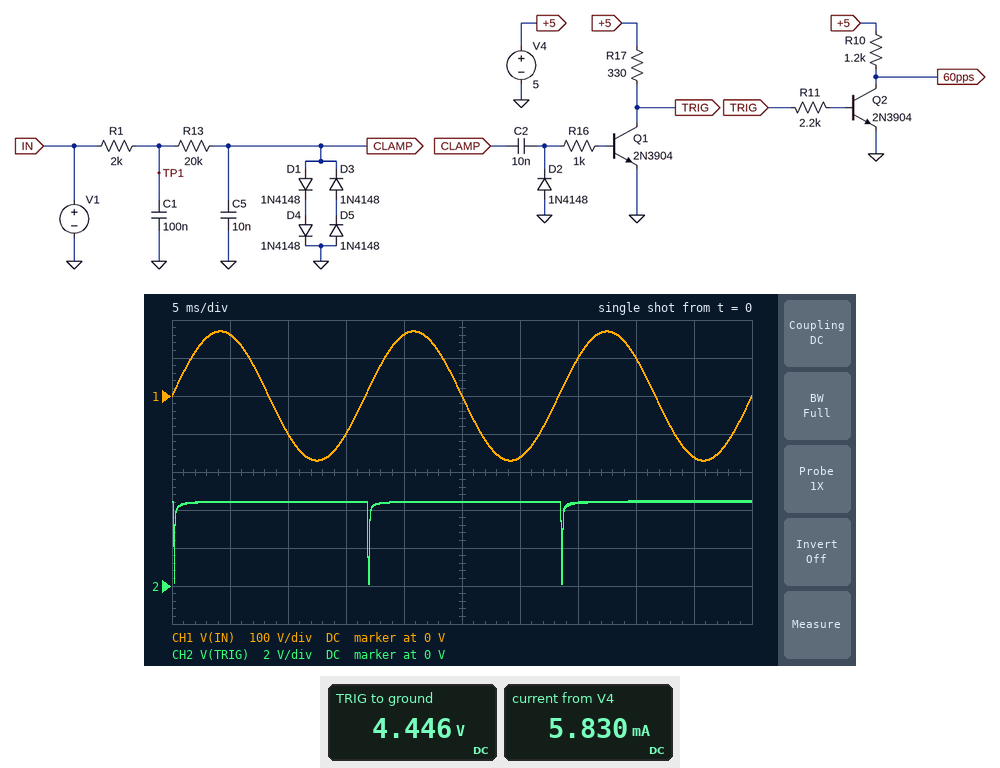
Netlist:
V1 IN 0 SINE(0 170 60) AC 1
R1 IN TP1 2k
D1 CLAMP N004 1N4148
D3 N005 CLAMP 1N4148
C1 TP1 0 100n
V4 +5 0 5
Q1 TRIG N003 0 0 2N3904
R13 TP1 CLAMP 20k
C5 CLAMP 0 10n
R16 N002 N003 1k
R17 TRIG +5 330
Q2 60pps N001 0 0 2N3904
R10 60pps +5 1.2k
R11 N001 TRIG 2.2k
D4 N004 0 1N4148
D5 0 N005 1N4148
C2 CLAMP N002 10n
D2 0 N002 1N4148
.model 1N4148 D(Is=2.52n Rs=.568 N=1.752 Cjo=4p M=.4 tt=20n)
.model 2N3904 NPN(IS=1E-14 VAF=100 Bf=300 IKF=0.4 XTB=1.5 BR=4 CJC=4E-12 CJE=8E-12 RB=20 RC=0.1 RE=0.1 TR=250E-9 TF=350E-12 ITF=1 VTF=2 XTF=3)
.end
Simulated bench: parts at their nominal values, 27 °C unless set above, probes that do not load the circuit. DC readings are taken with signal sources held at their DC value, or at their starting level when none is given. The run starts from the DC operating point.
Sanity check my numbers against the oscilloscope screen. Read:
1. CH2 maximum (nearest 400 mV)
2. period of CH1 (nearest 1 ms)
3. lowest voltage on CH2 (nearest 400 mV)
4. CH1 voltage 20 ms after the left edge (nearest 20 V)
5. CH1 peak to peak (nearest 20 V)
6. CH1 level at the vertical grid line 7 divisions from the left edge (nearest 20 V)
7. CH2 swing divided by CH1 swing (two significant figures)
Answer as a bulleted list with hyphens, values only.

- 4.4 V
- 17 ms
- 0 V
- 160 V
- 340 V
- 100 V
- 0.013
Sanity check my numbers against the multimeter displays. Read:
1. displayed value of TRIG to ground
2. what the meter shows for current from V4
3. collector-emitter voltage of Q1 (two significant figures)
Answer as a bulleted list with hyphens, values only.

- 4.446 V
- 5.830 mA
- 4.4 V
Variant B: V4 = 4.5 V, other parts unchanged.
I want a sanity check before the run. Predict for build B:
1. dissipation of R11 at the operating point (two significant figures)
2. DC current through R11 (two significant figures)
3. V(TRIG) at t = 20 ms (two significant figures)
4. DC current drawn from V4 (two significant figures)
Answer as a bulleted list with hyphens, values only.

- 4.8 mW
- 1.5 mA
- 4.0 V
- 5.2 mA
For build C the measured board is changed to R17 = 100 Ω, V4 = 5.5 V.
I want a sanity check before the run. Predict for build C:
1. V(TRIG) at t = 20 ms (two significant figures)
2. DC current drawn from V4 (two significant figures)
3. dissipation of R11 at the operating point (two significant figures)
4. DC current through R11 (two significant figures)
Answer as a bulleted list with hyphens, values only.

- 5.3 V
- 6.6 mA
- 9.3 mW
- 2.1 mA
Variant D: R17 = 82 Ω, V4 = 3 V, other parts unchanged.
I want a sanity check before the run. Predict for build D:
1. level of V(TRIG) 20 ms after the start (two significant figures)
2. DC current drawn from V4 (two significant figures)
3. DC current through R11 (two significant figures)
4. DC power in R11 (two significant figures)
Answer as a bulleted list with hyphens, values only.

- 2.9 V
- 3.5 mA
- 1.0 mA
- 2.2 mW
